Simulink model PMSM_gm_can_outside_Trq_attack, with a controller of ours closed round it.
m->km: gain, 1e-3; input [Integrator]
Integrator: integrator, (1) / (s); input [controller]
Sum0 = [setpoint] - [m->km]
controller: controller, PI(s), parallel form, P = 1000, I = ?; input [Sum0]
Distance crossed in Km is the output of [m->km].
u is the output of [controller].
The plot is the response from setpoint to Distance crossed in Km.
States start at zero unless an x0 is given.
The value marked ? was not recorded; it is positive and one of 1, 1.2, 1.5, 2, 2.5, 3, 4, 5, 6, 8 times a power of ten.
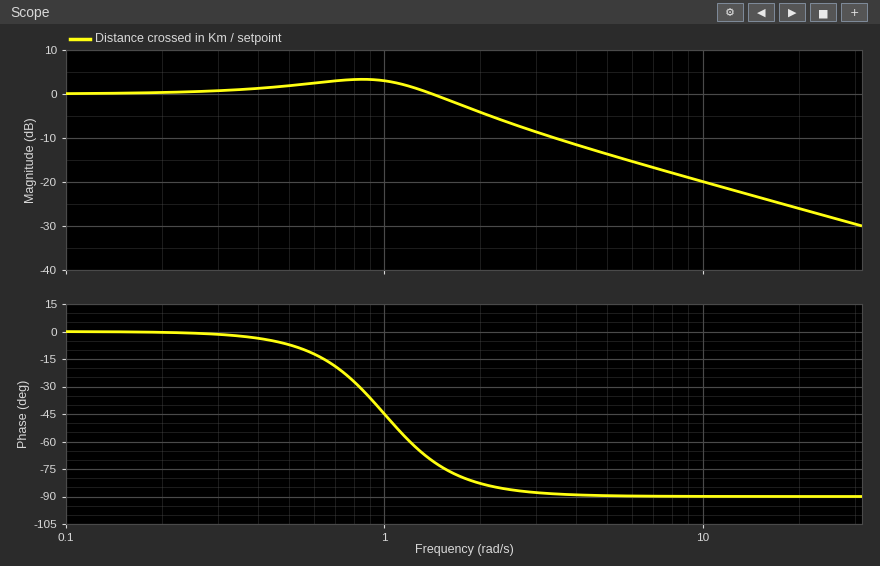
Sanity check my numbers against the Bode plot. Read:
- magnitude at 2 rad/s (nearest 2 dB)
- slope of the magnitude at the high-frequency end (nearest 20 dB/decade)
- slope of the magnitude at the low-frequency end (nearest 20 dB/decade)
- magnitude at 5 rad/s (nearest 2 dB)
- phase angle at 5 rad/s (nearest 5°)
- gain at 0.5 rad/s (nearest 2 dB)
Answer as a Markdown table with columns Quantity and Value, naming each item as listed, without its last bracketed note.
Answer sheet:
| Quantity | Value |
|---|---|
| magnitude at 2 rad/s | -4 dB |
| slope of the magnitude at the high-frequency end | -20 dB/decade |
| slope of the magnitude at the low-frequency end | 0 dB/decade |
| magnitude at 5 rad/s | -14 dB |
| phase angle at 5 rad/s | -90° |
| gain at 0.5 rad/s | 2 dB |
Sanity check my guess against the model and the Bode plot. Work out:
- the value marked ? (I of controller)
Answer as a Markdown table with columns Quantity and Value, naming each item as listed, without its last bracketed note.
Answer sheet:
| Quantity | Value |
|---|---|
| the value marked ? | 1000 |
